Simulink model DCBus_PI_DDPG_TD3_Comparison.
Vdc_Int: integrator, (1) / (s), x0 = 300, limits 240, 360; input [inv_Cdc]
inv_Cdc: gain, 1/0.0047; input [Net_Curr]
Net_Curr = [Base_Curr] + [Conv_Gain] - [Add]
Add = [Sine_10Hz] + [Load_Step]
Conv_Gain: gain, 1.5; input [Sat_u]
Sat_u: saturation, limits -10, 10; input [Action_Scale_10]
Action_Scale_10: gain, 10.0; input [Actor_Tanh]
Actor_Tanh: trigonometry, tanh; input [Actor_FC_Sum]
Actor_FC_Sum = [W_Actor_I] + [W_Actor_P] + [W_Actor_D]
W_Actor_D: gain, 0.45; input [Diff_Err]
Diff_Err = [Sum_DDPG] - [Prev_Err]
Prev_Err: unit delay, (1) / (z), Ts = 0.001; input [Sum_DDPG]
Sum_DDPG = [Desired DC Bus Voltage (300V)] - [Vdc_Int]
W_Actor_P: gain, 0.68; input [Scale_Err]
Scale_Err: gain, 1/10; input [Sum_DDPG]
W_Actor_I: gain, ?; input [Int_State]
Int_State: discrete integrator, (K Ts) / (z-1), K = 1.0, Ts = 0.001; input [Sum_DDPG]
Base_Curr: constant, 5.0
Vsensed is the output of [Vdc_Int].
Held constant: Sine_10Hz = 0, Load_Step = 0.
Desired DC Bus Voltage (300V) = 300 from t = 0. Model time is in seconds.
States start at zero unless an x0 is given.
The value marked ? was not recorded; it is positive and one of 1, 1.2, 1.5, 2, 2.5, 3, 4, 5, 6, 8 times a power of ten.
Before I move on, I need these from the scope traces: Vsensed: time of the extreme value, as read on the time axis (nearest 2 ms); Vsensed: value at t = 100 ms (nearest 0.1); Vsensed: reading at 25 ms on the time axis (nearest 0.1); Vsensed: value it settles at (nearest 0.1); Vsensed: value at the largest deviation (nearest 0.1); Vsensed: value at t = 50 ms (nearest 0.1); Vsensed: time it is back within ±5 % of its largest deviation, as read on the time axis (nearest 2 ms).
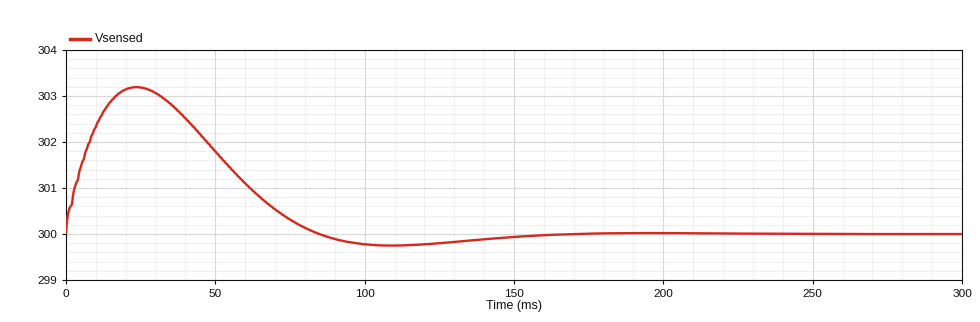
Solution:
24 ms
299.8
303.2
300.0
303.2
301.8
132 ms
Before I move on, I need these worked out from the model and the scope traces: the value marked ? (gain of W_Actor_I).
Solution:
2.5
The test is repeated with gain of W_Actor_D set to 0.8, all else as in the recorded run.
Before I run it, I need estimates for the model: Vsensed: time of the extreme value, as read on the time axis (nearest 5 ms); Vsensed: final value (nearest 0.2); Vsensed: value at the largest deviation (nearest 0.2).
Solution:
30 ms
300.0
302.8
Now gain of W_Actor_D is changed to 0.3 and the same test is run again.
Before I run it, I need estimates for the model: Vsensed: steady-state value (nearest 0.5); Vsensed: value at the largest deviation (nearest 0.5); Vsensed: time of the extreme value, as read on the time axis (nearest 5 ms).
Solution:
300.0
303.5
20 ms
